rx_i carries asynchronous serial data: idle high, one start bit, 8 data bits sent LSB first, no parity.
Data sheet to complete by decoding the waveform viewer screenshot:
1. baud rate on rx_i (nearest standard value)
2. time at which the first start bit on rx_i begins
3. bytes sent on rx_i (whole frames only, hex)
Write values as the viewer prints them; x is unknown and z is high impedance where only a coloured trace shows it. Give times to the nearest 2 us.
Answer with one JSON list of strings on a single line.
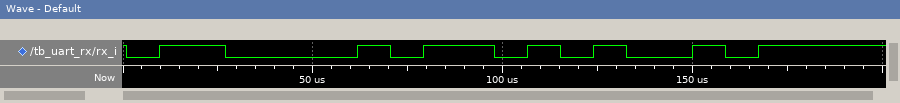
["115200 baud", "0 us", "43, A5"]
